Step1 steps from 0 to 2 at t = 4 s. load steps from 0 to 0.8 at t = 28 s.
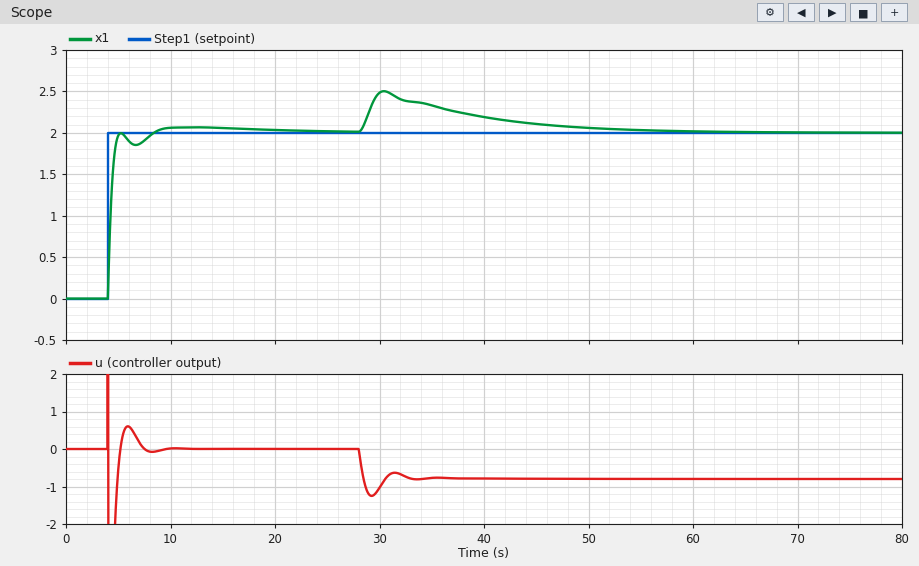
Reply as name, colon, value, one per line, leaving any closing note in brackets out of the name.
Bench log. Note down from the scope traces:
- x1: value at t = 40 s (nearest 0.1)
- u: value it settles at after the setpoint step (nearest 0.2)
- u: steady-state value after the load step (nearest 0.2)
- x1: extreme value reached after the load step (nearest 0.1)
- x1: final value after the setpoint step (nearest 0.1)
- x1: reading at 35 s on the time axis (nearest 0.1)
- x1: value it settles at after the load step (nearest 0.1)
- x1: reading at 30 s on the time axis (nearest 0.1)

x1: value at t = 40 s: 2.2
u: value it settles at after the setpoint step: 0.0
u: steady-state value after the load step: -0.8
x1: extreme value reached after the load step: 2.5
x1: final value after the setpoint step: 2.0
x1: reading at 35 s on the time axis: 2.3
x1: value it settles at after the load step: 2.0
x1: reading at 30 s on the time axis: 2.5
